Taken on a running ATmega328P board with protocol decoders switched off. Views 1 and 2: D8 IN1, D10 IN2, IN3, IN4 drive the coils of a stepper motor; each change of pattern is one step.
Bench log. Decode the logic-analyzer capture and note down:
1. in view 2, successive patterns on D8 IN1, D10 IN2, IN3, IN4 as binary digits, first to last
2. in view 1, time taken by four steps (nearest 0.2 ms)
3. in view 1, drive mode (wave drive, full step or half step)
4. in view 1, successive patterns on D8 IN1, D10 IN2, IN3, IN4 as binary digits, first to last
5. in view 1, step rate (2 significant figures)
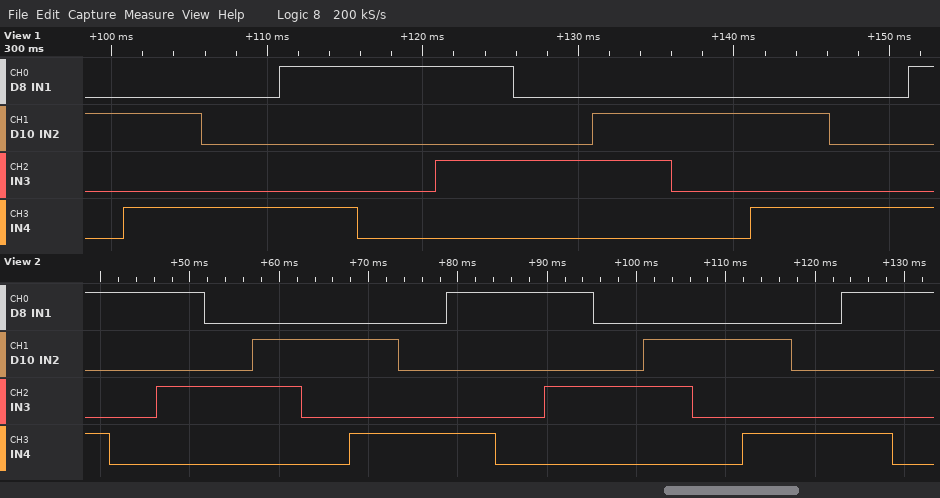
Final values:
1001 1000 1010 0010 0110 0100 0101 0001 1001 1000 1010 0010 0110 0100 0101 0001 1001 1000
20.0 ms
half step
0100 0101 0001 1001 1000 1010 0010 0110 0100 0101 0001 1001
200 steps/s
